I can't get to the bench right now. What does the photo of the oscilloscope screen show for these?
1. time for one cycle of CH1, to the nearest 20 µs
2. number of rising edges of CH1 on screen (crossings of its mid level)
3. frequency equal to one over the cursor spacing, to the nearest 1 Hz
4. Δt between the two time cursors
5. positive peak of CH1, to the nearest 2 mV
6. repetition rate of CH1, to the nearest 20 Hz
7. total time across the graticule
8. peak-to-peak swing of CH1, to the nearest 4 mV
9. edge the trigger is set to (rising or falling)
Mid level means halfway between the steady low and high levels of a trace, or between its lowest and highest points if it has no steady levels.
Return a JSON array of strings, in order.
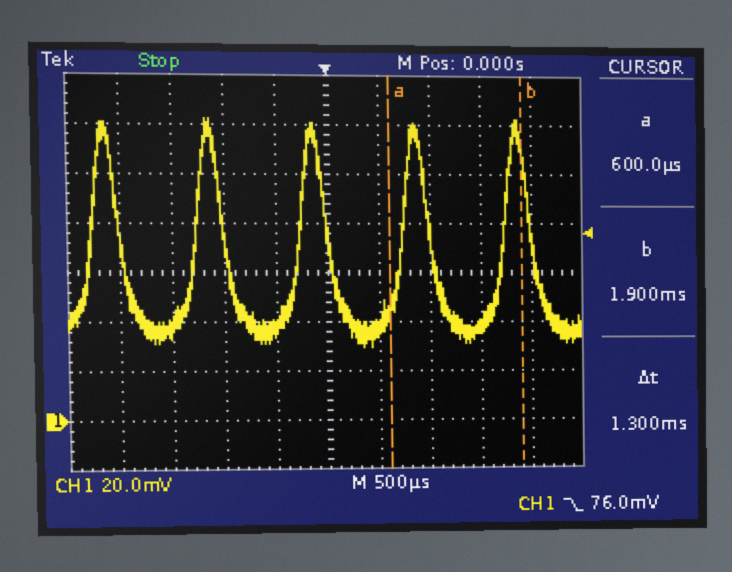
["1.00 ms", "5", "769 Hz", "1.3 ms", "122 mV", "1.00 kHz", "5 ms", "92 mV", "falling"]
